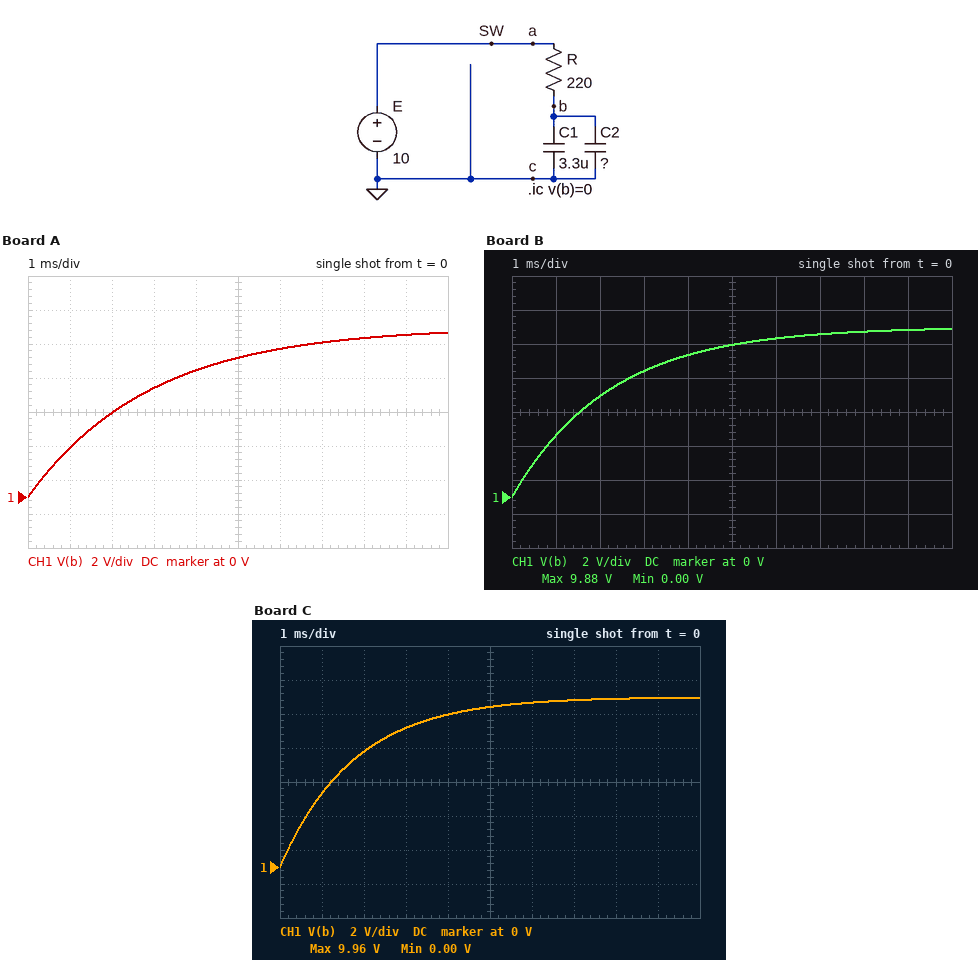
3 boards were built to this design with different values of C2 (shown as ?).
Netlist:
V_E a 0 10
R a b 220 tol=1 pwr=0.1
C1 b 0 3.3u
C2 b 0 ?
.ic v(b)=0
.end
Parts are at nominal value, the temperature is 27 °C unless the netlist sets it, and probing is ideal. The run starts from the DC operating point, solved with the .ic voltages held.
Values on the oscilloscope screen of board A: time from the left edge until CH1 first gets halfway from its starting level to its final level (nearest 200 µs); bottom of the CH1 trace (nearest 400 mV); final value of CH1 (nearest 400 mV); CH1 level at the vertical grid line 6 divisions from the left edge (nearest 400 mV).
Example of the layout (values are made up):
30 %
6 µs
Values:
2.0 ms
0 V
9.6 V
8.8 V
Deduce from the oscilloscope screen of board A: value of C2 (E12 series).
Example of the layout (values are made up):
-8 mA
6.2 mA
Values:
10 µF
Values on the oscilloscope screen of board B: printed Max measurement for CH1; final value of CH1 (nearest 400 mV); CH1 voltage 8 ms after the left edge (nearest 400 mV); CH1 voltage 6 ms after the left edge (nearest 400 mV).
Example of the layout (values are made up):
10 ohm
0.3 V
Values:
9.88 V
10.0 V
9.6 V
9.2 V
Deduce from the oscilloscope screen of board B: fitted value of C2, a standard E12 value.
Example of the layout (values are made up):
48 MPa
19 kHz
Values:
6.8 µF
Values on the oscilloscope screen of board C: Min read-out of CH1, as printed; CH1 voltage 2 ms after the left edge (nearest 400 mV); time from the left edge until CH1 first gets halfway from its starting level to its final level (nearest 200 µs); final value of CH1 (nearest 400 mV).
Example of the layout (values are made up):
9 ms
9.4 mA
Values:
0.00 V
6.8 V
1.2 ms
10.0 V
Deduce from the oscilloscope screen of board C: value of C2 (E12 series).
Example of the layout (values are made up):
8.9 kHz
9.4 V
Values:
4.7 µF
